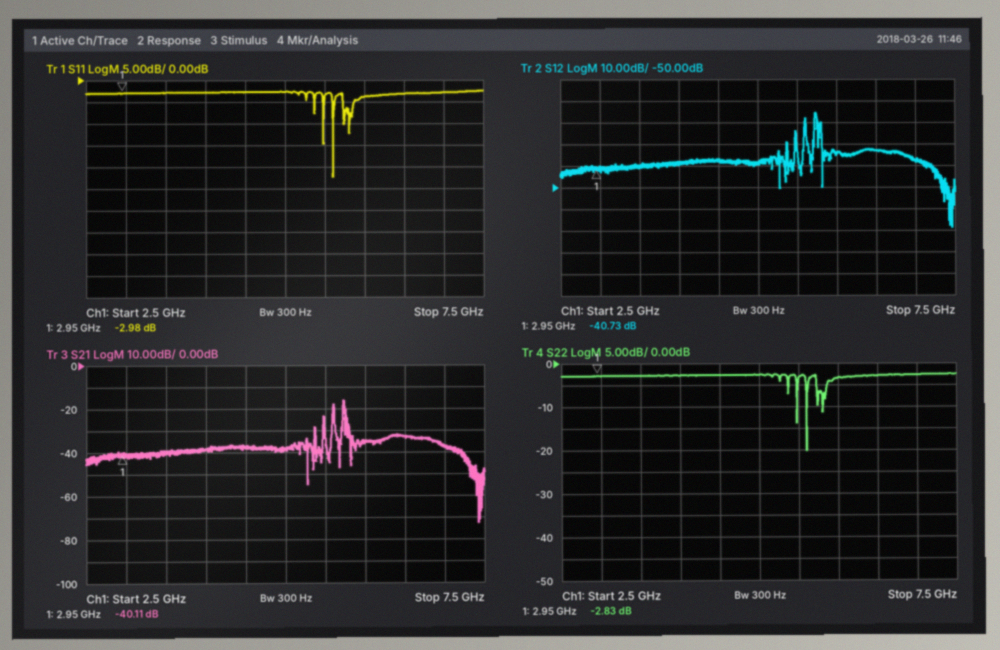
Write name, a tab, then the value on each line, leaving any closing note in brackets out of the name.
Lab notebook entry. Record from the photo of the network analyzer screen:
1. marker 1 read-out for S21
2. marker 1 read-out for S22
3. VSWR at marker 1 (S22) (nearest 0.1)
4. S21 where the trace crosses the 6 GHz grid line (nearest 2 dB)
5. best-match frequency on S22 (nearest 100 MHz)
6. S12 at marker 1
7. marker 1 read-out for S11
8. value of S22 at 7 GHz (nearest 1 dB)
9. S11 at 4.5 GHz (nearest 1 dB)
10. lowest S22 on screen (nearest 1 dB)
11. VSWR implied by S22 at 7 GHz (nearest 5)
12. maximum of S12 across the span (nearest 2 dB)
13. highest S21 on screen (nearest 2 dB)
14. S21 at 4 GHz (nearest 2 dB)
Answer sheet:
marker 1 read-out for S21	-40.11 dB
marker 1 read-out for S22	-2.83 dB
VSWR at marker 1 (S22)	6.2
S21 where the trace crosses the 6 GHz grid line	-36 dB
best-match frequency on S22	5.6 GHz
S12 at marker 1	-40.73 dB
marker 1 read-out for S11	-2.98 dB
value of S22 at 7 GHz	-3 dB
S11 at 4.5 GHz	-3 dB
lowest S22 on screen	-20 dB
VSWR implied by S22 at 7 GHz	5
maximum of S12 across the span	-16 dB
highest S21 on screen	-16 dB
S21 at 4 GHz	-38 dB
